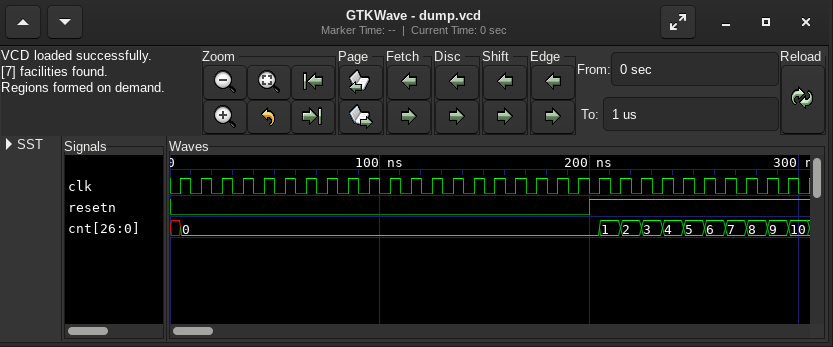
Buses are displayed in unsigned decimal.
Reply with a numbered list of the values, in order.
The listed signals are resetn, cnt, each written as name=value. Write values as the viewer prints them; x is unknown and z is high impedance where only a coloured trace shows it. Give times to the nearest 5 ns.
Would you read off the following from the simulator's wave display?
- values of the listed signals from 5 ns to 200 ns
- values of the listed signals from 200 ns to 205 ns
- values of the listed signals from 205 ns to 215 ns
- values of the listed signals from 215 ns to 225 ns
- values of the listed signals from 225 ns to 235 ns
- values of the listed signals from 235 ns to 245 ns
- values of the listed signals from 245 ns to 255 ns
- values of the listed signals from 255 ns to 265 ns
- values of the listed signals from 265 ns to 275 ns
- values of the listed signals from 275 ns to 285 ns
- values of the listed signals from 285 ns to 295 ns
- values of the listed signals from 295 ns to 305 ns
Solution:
1. resetn=0, cnt=0
2. resetn=1, cnt=0
3. resetn=1, cnt=1
4. resetn=1, cnt=2
5. resetn=1, cnt=3
6. resetn=1, cnt=4
7. resetn=1, cnt=5
8. resetn=1, cnt=6
9. resetn=1, cnt=7
10. resetn=1, cnt=8
11. resetn=1, cnt=9
12. resetn=1, cnt=10
